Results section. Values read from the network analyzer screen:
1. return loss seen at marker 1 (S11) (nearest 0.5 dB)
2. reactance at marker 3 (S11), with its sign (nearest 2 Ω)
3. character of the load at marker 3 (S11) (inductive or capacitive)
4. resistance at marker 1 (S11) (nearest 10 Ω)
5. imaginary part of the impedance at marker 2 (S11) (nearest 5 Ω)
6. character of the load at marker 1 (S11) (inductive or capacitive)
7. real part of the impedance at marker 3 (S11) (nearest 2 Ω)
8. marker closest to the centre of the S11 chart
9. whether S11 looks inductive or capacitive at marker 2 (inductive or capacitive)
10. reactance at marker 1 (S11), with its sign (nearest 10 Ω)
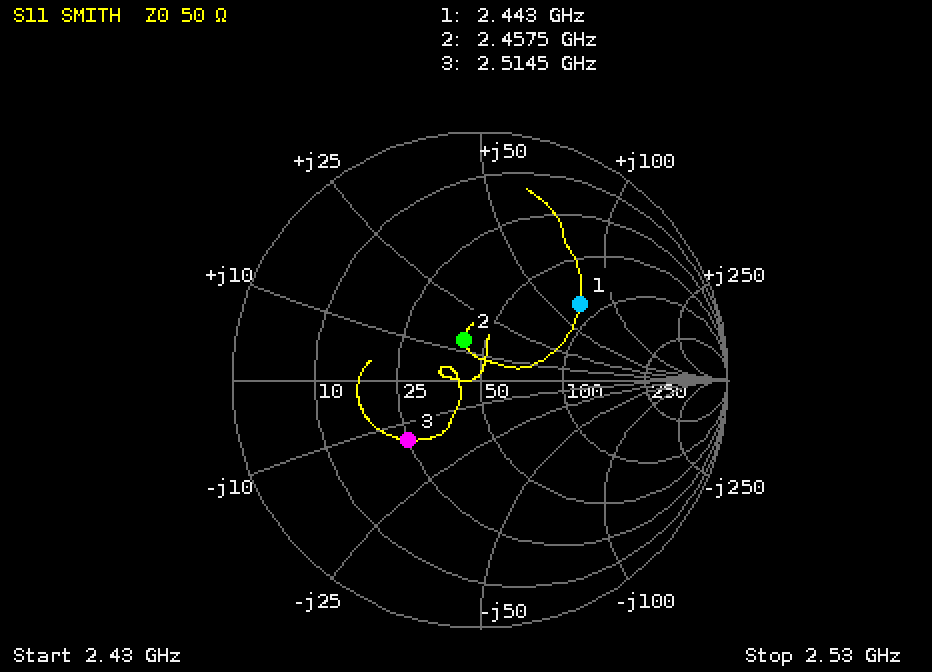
6.0 dB
-14 Ω
capacitive
80 Ω
+15 Ω
inductive
24 Ω
marker 2
inductive
+70 Ω
